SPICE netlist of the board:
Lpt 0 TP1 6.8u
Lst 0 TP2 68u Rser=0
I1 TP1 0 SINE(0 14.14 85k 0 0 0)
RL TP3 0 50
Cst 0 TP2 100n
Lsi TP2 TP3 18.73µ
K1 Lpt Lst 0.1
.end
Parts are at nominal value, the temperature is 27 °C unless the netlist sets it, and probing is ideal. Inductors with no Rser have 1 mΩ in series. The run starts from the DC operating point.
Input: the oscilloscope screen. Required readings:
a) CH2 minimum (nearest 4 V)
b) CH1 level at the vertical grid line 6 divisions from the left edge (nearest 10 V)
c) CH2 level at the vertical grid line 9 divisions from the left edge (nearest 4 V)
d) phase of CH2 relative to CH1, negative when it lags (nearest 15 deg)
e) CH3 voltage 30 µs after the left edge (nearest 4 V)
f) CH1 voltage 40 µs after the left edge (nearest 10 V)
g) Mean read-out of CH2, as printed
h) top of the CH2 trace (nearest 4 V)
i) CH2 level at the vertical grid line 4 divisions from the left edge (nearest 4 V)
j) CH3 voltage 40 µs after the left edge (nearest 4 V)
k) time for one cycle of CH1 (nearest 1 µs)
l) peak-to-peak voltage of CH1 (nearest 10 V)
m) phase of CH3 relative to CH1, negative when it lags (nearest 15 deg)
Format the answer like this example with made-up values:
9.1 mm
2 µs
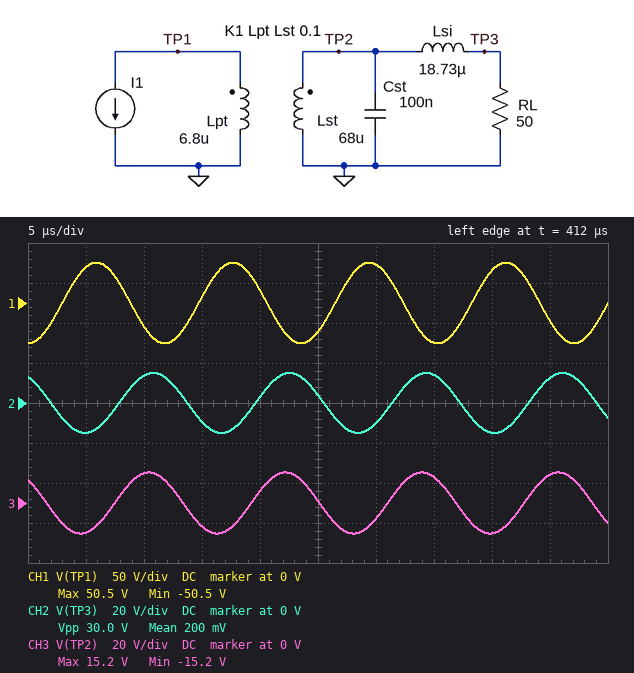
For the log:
-16 V
50 V
12 V
-150 deg
-8 V
40 V
200 mV
16 V
4 V
-16 V
12 µs
100 V
-135 deg
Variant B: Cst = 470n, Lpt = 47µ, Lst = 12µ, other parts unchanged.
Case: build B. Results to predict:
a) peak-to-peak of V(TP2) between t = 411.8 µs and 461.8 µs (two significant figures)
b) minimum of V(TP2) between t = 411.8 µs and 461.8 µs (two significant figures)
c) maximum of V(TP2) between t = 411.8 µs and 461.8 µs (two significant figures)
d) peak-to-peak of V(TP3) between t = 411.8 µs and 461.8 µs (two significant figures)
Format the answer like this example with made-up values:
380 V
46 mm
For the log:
60 V
-30 V
30 V
59 V
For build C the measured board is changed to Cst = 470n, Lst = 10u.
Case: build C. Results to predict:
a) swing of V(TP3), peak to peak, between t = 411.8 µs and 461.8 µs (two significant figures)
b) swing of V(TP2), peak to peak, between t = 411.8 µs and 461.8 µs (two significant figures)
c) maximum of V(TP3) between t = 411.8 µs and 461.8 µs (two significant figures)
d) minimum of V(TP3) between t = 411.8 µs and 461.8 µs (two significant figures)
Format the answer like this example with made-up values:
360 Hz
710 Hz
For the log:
36 V
37 V
18 V
-18 V
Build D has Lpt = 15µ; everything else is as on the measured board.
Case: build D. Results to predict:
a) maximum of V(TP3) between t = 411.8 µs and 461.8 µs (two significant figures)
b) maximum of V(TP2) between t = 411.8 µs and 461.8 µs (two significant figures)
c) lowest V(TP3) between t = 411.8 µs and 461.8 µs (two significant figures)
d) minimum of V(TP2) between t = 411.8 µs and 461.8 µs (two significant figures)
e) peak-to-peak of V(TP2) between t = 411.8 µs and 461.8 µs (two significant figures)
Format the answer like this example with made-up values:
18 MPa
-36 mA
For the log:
22 V
23 V
-22 V
-23 V
45 V
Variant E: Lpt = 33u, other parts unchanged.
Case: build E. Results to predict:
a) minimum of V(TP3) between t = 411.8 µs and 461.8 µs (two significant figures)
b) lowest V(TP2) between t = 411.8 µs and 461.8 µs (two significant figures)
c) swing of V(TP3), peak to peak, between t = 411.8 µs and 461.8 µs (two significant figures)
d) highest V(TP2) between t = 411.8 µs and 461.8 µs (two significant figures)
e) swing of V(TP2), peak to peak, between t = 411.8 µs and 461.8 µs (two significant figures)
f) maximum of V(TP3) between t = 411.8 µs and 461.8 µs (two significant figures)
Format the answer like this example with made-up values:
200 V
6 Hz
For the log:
-33 V
-34 V
66 V
34 V
67 V
33 V
